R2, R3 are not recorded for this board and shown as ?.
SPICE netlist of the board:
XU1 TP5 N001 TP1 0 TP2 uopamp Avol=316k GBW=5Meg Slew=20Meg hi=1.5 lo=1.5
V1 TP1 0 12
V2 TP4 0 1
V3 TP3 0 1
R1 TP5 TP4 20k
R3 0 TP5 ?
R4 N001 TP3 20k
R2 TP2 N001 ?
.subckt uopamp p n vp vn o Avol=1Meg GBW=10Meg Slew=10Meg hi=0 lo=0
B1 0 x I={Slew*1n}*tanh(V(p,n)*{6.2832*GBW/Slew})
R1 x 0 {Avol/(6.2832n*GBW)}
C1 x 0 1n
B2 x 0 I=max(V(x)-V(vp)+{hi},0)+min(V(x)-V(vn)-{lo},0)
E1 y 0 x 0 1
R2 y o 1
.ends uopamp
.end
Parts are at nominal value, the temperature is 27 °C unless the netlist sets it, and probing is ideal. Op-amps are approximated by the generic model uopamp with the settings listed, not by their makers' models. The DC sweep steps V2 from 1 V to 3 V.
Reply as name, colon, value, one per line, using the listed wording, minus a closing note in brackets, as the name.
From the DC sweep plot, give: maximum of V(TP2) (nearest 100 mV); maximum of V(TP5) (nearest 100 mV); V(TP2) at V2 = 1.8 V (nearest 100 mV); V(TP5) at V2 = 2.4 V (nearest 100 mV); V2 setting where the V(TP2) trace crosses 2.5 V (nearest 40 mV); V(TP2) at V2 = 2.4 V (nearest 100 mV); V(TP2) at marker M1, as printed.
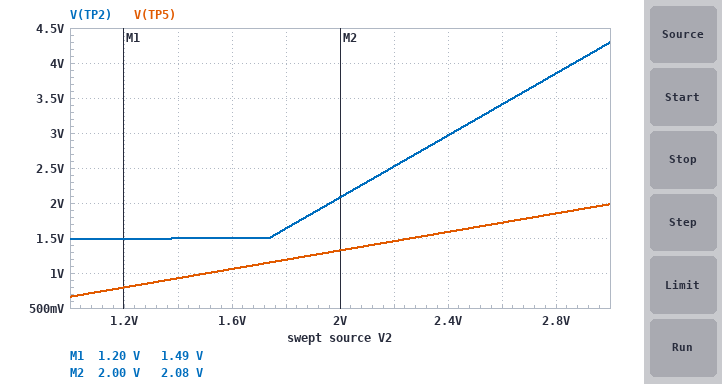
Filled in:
maximum of V(TP2): 4.3 V
maximum of V(TP5): 2.0 V
V(TP2) at V2 = 1.8 V: 1.6 V
V(TP5) at V2 = 2.4 V: 1.6 V
V2 setting where the V(TP2) trace crosses 2.5 V: 2.20 V
V(TP2) at V2 = 2.4 V: 3.0 V
V(TP2) at marker M1, as printed: 1.49 V
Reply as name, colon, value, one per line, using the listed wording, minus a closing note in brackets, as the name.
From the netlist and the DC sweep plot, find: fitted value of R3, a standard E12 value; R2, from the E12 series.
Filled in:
fitted value of R3, a standard E12 value: 39 kΩ
R2, from the E12 series: 47 kΩ
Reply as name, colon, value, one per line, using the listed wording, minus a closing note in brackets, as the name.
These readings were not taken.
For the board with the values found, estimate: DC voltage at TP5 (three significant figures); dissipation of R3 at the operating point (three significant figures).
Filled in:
DC voltage at TP5: 661 mV
dissipation of R3 at the operating point: 11.2 µW
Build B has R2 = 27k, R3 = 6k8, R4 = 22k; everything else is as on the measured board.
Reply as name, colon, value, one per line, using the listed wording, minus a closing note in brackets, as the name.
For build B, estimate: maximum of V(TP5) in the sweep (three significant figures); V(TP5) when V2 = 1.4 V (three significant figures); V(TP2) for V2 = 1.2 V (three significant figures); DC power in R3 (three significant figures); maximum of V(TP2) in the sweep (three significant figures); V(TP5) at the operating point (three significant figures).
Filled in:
maximum of V(TP5) in the sweep: 761 mV
V(TP5) when V2 = 1.4 V: 355 mV
V(TP2) for V2 = 1.2 V: 1.48 V
DC power in R3: 9.47 µW
maximum of V(TP2) in the sweep: 1.49 V
V(TP5) at the operating point: 254 mV
